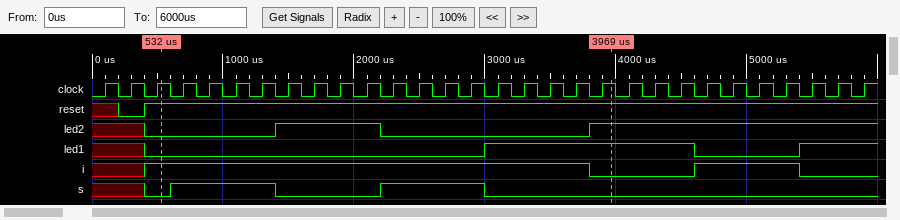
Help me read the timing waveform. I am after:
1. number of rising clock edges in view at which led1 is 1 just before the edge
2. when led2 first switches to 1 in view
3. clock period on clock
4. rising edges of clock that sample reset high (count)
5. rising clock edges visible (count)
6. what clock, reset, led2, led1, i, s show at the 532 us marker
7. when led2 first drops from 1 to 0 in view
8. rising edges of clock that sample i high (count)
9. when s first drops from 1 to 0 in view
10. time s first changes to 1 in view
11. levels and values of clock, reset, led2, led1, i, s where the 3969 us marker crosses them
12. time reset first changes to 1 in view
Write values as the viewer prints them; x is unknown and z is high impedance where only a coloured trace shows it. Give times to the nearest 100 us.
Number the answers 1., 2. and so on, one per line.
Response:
1. 11
2. 1400 us
3. 200 us
4. 28
5. 30
6. clock=1, reset=1, led2=0, led1=0, i=1, s=0
7. 2200 us
8. 21
9. 1400 us
10. 600 us
11. clock=1, reset=1, led2=1, led1=1, i=0, s=0
12. 400 us
